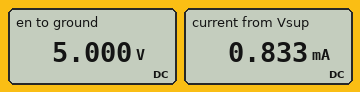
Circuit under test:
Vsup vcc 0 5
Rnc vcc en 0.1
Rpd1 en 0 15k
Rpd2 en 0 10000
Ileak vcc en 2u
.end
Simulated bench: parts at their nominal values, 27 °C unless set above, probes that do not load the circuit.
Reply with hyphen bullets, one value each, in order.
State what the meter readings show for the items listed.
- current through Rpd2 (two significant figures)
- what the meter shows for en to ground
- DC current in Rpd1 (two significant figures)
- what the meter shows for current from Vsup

- 500 µA
- 5.000 V
- 330 µA
- 0.833 mA
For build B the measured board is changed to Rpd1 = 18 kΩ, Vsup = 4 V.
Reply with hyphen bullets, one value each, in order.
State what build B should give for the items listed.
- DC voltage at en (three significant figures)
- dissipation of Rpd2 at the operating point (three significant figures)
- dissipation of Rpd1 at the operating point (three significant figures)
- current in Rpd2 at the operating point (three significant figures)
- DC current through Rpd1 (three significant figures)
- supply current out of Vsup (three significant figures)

- 4.00 V
- 1.60 mW
- 889 µW
- 400 µA
- 222 µA
- 622 µA
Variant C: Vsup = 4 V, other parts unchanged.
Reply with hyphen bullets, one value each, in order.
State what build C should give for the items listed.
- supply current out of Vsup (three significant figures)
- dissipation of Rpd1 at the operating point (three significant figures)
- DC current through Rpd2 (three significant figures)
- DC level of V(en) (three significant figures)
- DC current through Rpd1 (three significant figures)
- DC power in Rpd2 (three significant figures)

- 667 µA
- 1.07 mW
- 400 µA
- 4.00 V
- 267 µA
- 1.60 mW
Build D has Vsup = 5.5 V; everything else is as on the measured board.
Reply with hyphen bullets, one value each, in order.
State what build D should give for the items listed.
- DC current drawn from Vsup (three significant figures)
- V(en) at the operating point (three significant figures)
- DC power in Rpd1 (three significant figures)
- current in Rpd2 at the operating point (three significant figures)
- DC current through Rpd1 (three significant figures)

- 917 µA
- 5.50 V
- 2.02 mW
- 550 µA
- 367 µA
